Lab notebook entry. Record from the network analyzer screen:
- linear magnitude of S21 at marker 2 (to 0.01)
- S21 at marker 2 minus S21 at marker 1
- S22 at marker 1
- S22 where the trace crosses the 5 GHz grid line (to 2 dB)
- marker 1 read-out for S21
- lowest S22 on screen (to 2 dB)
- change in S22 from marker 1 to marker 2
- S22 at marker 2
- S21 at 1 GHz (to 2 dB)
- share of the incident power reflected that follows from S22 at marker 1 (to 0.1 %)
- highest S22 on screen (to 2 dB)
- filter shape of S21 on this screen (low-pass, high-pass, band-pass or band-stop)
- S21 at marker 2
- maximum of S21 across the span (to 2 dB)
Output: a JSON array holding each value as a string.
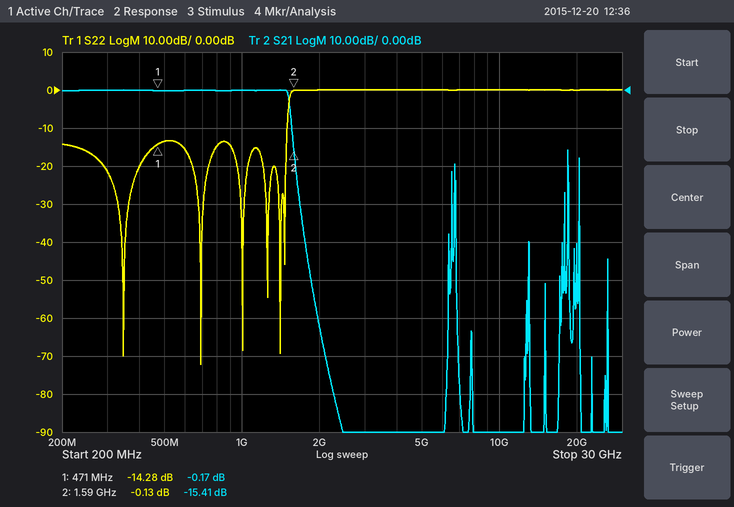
["0.17", "-15.24 dB", "-14.28 dB", "0 dB", "-0.17 dB", "-72 dB", "14.15 dB", "-0.13 dB", "0 dB", "3.7 %", "0 dB", "low-pass", "-15.41 dB", "0 dB"]
